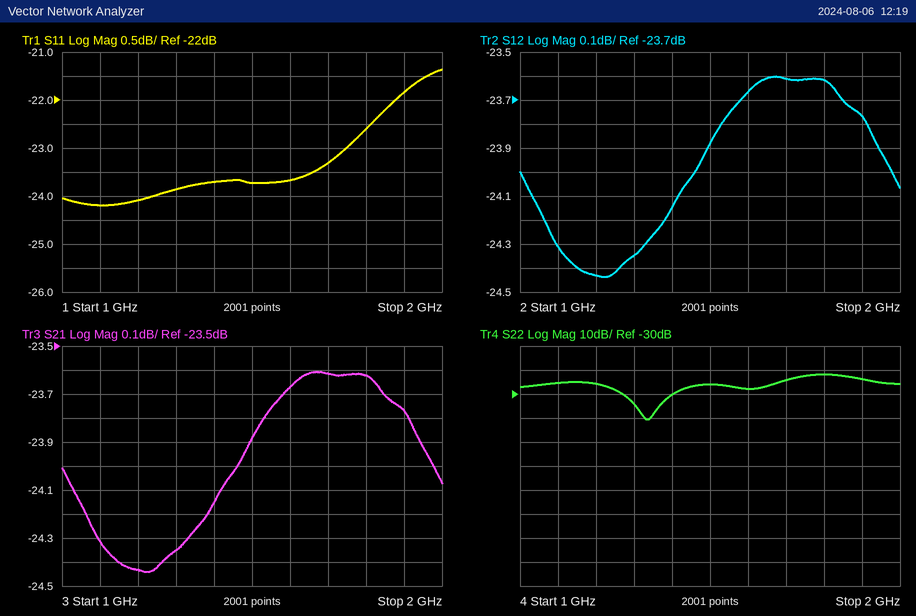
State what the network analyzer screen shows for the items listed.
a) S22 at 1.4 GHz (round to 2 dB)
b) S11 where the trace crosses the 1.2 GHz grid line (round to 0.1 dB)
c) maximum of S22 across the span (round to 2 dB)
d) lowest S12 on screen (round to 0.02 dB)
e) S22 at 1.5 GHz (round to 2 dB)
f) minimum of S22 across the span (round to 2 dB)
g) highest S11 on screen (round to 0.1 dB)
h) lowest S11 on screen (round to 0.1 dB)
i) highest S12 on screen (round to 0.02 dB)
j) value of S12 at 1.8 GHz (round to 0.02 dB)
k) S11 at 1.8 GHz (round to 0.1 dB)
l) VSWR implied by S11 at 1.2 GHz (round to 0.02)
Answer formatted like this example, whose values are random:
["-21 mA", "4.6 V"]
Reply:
["-30 dB", "-24.1 dB", "-22 dB", "-24.44 dB", "-26 dB", "-40 dB", "-21.4 dB", "-24.2 dB", "-23.60 dB", "-23.62 dB", "-22.6 dB", "1.14"]
